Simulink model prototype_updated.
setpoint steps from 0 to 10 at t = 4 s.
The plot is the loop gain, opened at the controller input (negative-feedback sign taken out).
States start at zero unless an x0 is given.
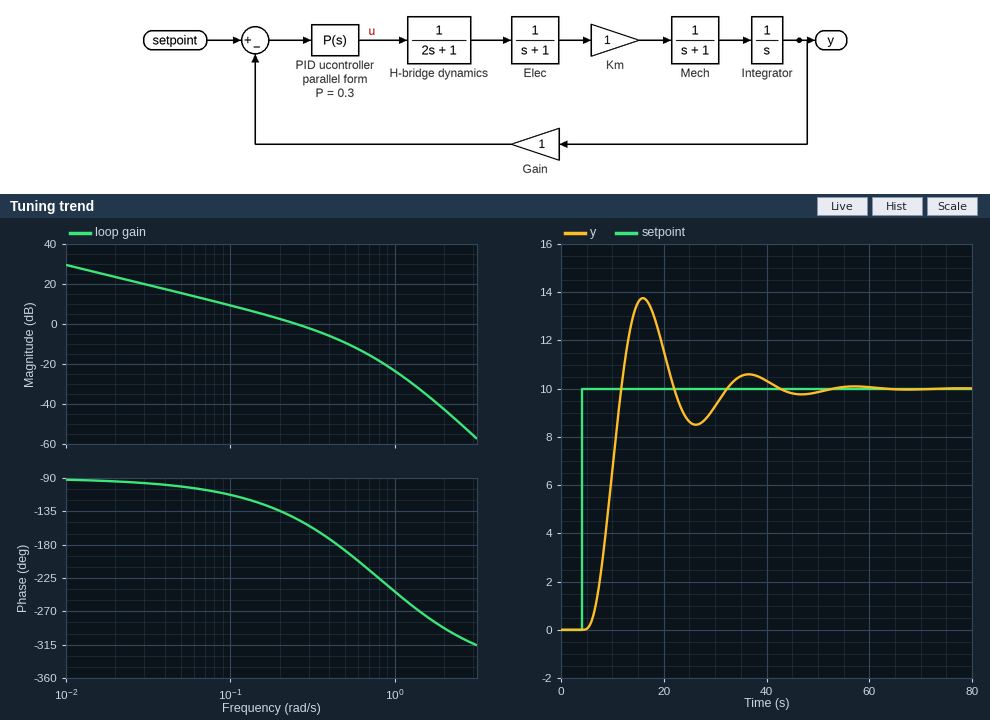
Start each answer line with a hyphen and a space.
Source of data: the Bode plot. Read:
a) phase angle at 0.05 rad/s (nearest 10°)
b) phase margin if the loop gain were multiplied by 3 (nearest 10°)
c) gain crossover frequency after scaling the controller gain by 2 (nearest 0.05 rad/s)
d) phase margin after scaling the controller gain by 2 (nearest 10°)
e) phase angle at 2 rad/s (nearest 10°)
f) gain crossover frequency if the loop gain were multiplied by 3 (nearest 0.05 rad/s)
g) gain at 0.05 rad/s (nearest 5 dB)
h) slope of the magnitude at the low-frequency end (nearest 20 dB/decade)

- -100°
- -10°
- 0.40 rad/s
- 10°
- -290°
- 0.50 rad/s
- 15 dB
- -20 dB/decade
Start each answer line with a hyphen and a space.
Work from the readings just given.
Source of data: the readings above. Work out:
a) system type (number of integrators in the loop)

- 1
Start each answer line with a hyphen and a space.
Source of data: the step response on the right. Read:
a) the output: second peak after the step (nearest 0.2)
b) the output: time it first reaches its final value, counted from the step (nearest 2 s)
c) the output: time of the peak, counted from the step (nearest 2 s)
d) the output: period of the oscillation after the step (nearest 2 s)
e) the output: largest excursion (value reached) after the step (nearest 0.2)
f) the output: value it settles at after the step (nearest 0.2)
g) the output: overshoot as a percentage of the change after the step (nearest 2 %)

- 10.6
- 8 s
- 12 s
- 20 s
- 13.8
- 10.0
- 38 %
